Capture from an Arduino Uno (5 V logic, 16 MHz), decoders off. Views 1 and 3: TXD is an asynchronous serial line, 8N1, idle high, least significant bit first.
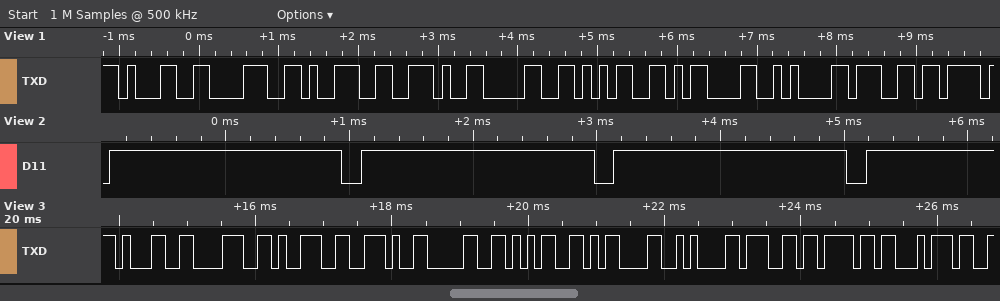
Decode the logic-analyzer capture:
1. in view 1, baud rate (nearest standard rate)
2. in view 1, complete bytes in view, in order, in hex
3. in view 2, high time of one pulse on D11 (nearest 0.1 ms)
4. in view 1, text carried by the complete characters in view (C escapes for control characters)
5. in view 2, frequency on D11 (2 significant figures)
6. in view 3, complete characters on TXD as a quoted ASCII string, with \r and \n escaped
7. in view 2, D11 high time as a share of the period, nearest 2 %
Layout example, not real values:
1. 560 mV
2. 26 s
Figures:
1. 9600 baud
2. 31 38 39 2E 30 35 0D 0A 67
3. 1.9 ms
4. "189.05\r\ng"
5. 490 Hz
6. "189.05\r\ngot"
7. 92 %
